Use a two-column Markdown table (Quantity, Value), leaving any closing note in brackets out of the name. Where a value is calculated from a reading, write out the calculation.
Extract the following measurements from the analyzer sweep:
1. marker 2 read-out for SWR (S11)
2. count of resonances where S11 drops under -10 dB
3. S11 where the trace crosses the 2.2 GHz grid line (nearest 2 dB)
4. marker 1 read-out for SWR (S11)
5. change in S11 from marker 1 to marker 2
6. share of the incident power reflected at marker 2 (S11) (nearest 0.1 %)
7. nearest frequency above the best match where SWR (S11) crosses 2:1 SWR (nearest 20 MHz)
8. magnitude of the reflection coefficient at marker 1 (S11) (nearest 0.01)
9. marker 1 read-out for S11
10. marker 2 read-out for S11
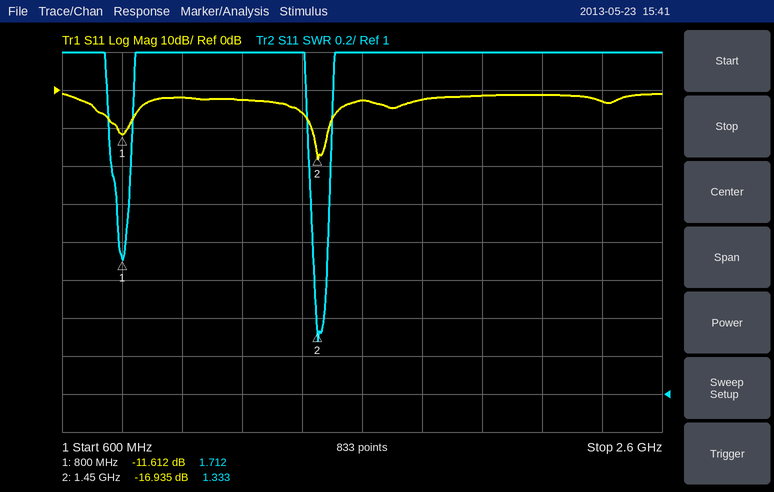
| Quantity | Value |
|---|---|
| marker 2 read-out for SWR | 1.333 |
| count of resonances where S11 drops under -10 dB | 2 |
| S11 where the trace crosses the 2.2 GHz grid line | -2 dB |
| marker 1 read-out for SWR | 1.712 |
| change in S11 from marker 1 to marker 2 | -16.935 − (-11.612) = -5.323 dB |
| share of the incident power reflected at marker 2 (S11) | 10^(-16.935/10) ≈ 2.0 % |
| nearest frequency above the best match where SWR (S11) crosses 2:1 SWR | 1.50 GHz |
| magnitude of the reflection coefficient at marker 1 (S11) | 10^(-11.612/20) ≈ 0.26 |
| marker 1 read-out for S11 | -11.612 dB |
| marker 2 read-out for S11 | -16.935 dB |
